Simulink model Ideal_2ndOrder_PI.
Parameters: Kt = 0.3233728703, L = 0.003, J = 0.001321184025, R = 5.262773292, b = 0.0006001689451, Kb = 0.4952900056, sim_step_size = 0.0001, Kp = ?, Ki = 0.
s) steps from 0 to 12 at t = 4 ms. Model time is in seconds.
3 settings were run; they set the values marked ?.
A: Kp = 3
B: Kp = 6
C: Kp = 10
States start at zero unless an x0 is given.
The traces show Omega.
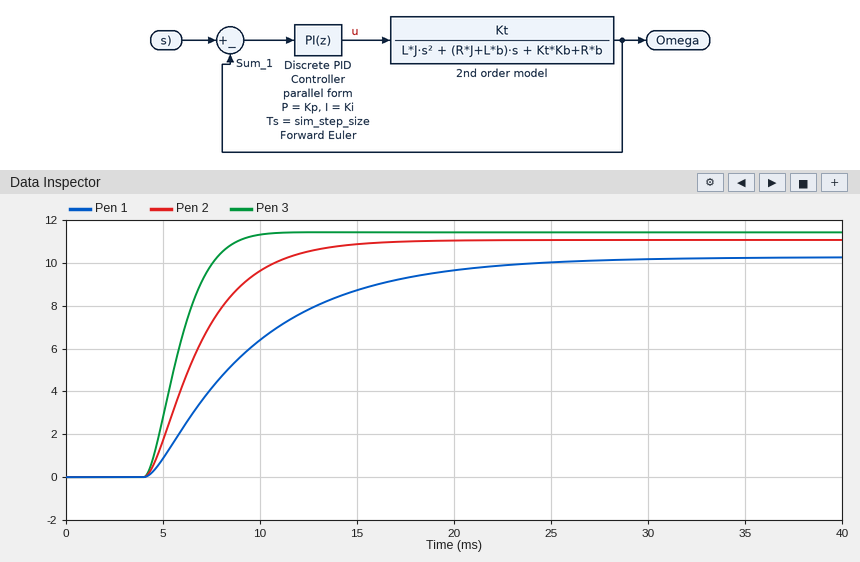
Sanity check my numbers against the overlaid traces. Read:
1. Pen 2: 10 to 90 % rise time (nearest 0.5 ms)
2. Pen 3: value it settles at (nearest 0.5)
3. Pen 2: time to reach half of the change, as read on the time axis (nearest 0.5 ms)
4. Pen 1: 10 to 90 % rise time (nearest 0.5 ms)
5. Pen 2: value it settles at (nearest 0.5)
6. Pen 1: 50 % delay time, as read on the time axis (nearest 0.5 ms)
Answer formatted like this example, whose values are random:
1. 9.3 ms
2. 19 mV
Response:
1. 6.0 ms
2. 11.5
3. 6.5 ms
4. 12.0 ms
5. 11.0
6. 8.5 ms
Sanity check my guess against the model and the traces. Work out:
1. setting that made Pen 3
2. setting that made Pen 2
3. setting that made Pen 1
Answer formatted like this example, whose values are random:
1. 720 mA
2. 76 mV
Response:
1. C
2. B
3. A
